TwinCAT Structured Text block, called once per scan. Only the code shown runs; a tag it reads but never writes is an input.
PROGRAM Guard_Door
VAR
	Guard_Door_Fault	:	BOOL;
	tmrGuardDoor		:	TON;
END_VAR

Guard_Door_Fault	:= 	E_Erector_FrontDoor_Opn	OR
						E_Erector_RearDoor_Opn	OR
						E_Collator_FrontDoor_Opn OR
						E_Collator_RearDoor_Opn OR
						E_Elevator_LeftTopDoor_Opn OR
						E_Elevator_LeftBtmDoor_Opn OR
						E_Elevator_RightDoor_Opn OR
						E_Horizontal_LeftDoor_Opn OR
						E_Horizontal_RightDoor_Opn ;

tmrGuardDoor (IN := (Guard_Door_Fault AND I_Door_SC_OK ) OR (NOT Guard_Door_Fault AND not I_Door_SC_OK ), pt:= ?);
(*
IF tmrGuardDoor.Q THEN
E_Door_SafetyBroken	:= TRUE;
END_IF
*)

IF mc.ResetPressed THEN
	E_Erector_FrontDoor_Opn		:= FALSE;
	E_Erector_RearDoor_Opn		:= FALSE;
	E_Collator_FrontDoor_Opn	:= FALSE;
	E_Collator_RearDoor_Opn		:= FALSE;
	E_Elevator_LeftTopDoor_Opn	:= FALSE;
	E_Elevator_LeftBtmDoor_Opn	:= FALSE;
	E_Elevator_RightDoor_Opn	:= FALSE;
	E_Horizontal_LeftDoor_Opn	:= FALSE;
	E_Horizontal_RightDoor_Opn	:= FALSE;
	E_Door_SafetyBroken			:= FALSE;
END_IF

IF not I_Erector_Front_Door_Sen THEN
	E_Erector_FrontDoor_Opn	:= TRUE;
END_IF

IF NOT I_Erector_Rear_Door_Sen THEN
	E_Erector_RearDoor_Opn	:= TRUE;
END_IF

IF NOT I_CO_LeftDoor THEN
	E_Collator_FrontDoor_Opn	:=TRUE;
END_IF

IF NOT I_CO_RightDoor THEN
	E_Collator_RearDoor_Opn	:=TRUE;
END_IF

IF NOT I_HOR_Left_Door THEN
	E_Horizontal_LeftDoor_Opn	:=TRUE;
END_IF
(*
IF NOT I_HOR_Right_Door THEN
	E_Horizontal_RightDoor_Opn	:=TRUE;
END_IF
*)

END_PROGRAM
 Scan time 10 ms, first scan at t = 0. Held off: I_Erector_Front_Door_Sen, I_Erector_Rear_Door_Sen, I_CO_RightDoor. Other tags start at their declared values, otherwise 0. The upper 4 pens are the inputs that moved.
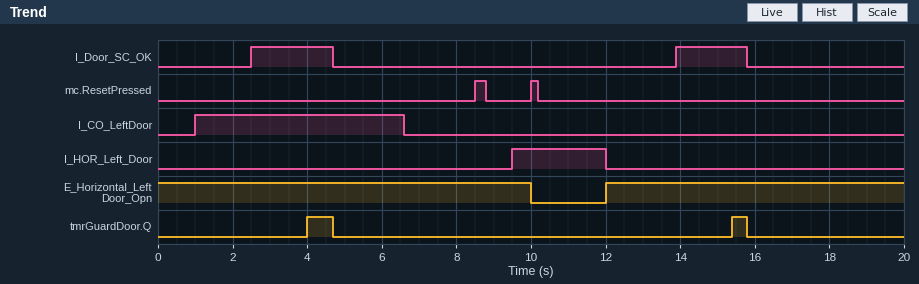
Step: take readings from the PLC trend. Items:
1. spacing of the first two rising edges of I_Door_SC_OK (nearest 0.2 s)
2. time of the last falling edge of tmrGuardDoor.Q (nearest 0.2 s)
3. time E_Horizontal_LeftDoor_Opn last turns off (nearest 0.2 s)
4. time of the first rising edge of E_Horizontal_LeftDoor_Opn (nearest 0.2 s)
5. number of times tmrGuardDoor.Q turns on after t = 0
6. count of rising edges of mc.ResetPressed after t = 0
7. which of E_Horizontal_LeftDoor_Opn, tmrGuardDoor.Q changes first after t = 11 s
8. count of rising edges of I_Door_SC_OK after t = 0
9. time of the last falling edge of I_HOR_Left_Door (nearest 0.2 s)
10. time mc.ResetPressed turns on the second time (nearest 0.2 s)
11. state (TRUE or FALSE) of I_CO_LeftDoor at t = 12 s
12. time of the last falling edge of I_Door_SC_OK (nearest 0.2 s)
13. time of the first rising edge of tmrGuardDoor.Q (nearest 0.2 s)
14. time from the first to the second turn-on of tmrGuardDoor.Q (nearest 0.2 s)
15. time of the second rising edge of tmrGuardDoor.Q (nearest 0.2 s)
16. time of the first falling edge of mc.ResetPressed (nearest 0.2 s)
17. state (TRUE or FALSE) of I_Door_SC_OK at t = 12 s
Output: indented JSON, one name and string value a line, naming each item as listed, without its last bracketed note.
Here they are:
{
  "spacing of the first two rising edges of I_Door_SC_OK": "11.4 s",
  "time of the last falling edge of tmrGuardDoor.Q": "15.8 s",
  "time E_Horizontal_LeftDoor_Opn last turns off": "10.0 s",
  "time of the first rising edge of E_Horizontal_LeftDoor_Opn": "12.0 s",
  "number of times tmrGuardDoor.Q turns on after t = 0": "2",
  "count of rising edges of mc.ResetPressed after t = 0": "2",
  "which of E_Horizontal_LeftDoor_Opn, tmrGuardDoor.Q changes first after t = 11 s": "E_Horizontal_LeftDoor_Opn",
  "count of rising edges of I_Door_SC_OK after t = 0": "2",
  "time of the last falling edge of I_HOR_Left_Door": "12.0 s",
  "time mc.ResetPressed turns on the second time": "10.0 s",
  "state (TRUE or FALSE) of I_CO_LeftDoor at t = 12 s": "FALSE",
  "time of the last falling edge of I_Door_SC_OK": "15.8 s",
  "time of the first rising edge of tmrGuardDoor.Q": "4.0 s",
  "time from the first to the second turn-on of tmrGuardDoor.Q": "11.4 s",
  "time of the second rising edge of tmrGuardDoor.Q": "15.4 s",
  "time of the first falling edge of mc.ResetPressed": "8.8 s",
  "state (TRUE or FALSE) of I_Door_SC_OK at t = 12 s": "FALSE"
}
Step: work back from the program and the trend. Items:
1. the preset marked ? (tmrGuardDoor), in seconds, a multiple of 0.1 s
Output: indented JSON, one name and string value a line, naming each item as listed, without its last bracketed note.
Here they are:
{
  "the preset marked ? (tmrGuardDoor), in seconds, a multiple of 0.1 s": "1.5 s"
}
